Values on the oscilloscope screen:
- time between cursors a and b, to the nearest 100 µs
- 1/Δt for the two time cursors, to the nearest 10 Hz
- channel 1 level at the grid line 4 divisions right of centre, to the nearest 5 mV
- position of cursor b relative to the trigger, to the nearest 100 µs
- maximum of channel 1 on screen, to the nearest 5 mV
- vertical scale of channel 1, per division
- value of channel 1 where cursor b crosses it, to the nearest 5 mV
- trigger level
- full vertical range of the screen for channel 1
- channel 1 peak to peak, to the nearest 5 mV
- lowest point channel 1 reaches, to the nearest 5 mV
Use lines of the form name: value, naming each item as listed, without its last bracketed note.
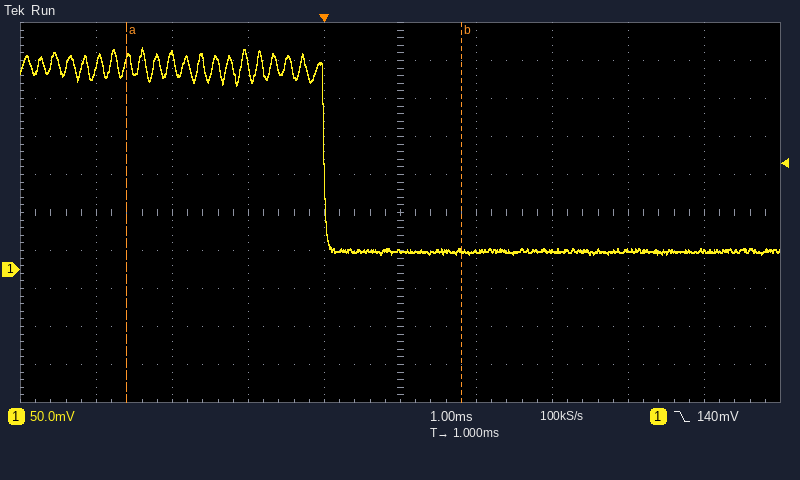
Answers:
time between cursors a and b, to the nearest 100 µs: 4.4 ms
1/Δt for the two time cursors, to the nearest 10 Hz: 230 Hz
channel 1 level at the grid line 4 divisions right of centre, to the nearest 5 mV: 25 mV
position of cursor b relative to the trigger, to the nearest 100 µs: +1.8 ms
maximum of channel 1 on screen, to the nearest 5 mV: 290 mV
vertical scale of channel 1, per division: 50 mV
value of channel 1 where cursor b crosses it, to the nearest 5 mV: 25 mV
trigger level: 140 mV
full vertical range of the screen for channel 1: 500 mV
channel 1 peak to peak, to the nearest 5 mV: 270 mV
lowest point channel 1 reaches, to the nearest 5 mV: 20 mV
